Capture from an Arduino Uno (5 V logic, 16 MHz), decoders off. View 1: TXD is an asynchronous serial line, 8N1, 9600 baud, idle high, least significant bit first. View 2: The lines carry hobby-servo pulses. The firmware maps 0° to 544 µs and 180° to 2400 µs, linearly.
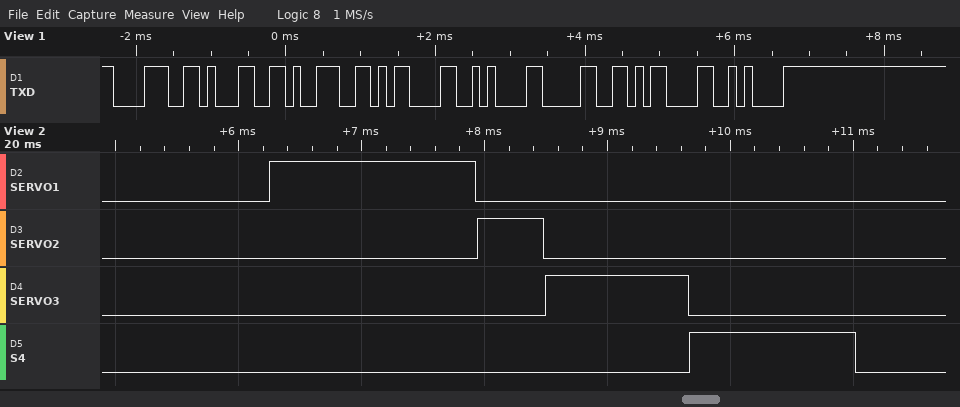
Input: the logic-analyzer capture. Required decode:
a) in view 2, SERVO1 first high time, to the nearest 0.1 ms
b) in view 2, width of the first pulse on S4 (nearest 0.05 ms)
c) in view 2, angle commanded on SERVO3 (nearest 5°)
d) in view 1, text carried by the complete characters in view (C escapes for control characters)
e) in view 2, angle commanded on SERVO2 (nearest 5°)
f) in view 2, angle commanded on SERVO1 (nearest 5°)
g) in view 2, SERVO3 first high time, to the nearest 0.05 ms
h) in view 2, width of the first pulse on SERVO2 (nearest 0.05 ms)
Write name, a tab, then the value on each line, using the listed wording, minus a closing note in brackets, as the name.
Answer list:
in view 2, SERVO1 first high time, to the nearest 0.1 ms	1.7 ms
in view 2, width of the first pulse on S4	1.35 ms
in view 2, angle commanded on SERVO3	60°
in view 1, text carried by the complete characters in view	"819\r\n0\r\n"
in view 2, angle commanded on SERVO2	0°
in view 2, angle commanded on SERVO1	110°
in view 2, SERVO3 first high time, to the nearest 0.05 ms	1.15 ms
in view 2, width of the first pulse on SERVO2	0.55 ms
